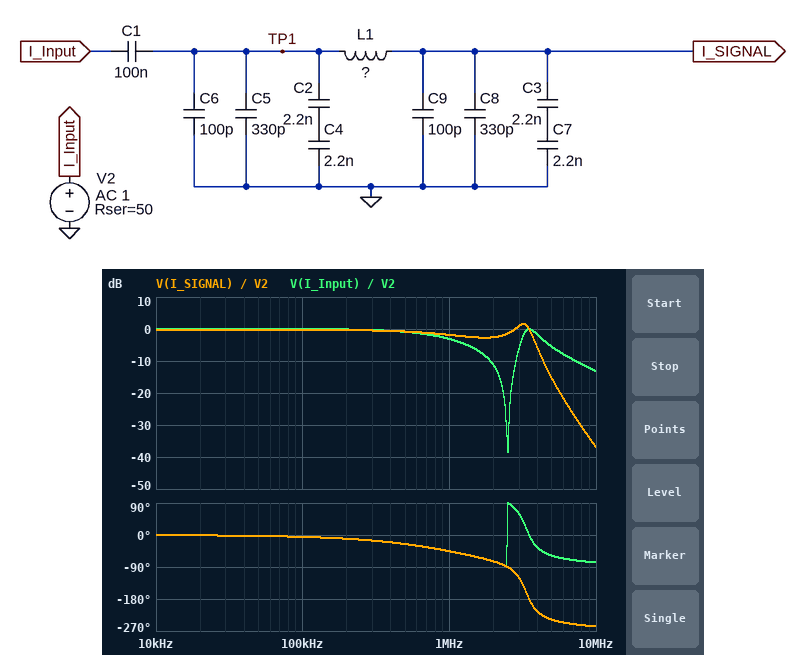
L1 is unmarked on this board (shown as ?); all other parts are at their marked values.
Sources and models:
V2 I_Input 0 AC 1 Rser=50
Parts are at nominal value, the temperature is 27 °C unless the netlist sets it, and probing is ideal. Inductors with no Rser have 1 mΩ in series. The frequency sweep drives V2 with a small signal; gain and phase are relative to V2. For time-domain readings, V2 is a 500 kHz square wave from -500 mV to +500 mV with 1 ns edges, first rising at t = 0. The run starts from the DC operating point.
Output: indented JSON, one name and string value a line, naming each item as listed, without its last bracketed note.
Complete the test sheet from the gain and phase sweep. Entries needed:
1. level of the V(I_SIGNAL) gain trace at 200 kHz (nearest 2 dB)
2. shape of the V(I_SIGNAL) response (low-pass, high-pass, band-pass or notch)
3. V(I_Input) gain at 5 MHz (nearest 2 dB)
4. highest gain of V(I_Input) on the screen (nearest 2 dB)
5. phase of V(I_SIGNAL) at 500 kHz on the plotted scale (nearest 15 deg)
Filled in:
{
  "level of the V(I_SIGNAL) gain trace at 200 kHz": "0 dB",
  "shape of the V(I_SIGNAL) response": "low-pass",
  "V(I_Input) gain at 5 MHz": "-6 dB",
  "highest gain of V(I_Input) on the screen": "0 dB",
  "phase of V(I_SIGNAL) at 500 kHz on the plotted scale": "-30 deg"
}
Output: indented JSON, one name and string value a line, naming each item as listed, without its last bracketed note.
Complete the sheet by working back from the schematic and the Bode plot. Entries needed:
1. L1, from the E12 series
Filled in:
{
  "L1, from the E12 series": "2.7 µH"
}
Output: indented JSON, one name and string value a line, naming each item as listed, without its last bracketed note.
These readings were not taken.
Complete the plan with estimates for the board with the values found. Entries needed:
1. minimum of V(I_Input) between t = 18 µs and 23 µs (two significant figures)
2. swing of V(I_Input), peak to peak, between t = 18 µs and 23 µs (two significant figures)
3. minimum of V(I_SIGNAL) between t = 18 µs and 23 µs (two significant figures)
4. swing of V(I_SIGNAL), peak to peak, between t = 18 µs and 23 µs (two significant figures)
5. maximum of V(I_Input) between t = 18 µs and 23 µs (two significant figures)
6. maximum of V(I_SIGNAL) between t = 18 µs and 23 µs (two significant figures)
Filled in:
{
  "minimum of V(I_Input) between t = 18 µs and 23 µs": "-540 mV",
  "swing of V(I_Input), peak to peak, between t = 18 µs and 23 µs": "1.1 V",
  "minimum of V(I_SIGNAL) between t = 18 µs and 23 µs": "-55 mV",
  "swing of V(I_SIGNAL), peak to peak, between t = 18 µs and 23 µs": "1.1 V",
  "maximum of V(I_Input) between t = 18 µs and 23 µs": "540 mV",
  "maximum of V(I_SIGNAL) between t = 18 µs and 23 µs": "1.0 V"
}
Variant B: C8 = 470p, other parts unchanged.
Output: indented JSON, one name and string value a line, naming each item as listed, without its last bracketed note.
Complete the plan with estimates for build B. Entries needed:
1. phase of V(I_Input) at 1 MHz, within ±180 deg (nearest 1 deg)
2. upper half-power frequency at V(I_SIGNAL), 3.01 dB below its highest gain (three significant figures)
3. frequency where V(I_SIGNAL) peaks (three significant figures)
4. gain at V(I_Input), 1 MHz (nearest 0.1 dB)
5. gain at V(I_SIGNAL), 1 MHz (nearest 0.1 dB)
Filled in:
{
  "phase of V(I_Input) at 1 MHz, within ±180 deg": "-47 deg",
  "upper half-power frequency at V(I_SIGNAL), 3.01 dB below its highest gain": "3.55 MHz",
  "frequency where V(I_SIGNAL) peaks": "3.11 MHz",
  "gain at V(I_Input), 1 MHz": "-3.4 dB",
  "gain at V(I_SIGNAL), 1 MHz": "-2.0 dB"
}
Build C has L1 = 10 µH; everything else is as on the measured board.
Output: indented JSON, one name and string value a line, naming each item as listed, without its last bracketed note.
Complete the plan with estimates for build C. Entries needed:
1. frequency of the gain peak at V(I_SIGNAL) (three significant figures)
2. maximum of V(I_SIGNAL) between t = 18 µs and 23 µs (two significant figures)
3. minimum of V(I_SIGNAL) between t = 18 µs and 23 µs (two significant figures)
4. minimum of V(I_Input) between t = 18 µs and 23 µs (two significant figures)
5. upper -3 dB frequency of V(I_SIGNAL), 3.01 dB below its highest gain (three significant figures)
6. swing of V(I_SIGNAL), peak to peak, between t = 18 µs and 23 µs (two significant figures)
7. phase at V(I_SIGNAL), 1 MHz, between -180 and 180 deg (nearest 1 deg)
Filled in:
{
  "frequency of the gain peak at V(I_SIGNAL)": "1.44 MHz",
  "maximum of V(I_SIGNAL) between t = 18 µs and 23 µs": "1.3 V",
  "minimum of V(I_SIGNAL) between t = 18 µs and 23 µs": "-370 mV",
  "minimum of V(I_Input) between t = 18 µs and 23 µs": "-660 mV",
  "upper -3 dB frequency of V(I_SIGNAL), 3.01 dB below its highest gain": "1.72 MHz",
  "swing of V(I_SIGNAL), peak to peak, between t = 18 µs and 23 µs": "1.7 V",
  "phase at V(I_SIGNAL), 1 MHz, between -180 and 180 deg": "-58 deg"
}
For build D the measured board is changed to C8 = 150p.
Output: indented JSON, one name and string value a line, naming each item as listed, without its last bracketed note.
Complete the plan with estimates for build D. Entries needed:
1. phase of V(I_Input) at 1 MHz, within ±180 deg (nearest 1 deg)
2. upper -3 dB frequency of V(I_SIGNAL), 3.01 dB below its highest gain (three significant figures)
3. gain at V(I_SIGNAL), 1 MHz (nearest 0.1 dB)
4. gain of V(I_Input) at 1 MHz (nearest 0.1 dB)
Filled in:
{
  "phase of V(I_Input) at 1 MHz, within ±180 deg": "-43 deg",
  "upper -3 dB frequency of V(I_SIGNAL), 3.01 dB below its highest gain": "3.75 MHz",
  "gain at V(I_SIGNAL), 1 MHz": "-1.7 dB",
  "gain of V(I_Input) at 1 MHz": "-2.8 dB"
}
